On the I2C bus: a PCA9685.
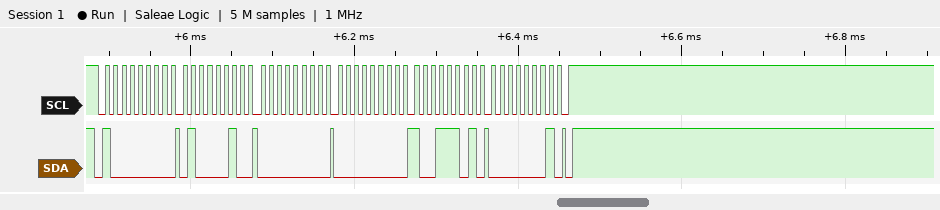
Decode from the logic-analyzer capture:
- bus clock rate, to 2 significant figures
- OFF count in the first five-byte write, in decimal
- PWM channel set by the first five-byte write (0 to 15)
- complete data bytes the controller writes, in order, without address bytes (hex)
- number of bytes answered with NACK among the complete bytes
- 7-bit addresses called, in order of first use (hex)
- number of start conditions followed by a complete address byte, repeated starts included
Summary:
100 kHz
413
15
42 00 00 9D 01
0
0x40
1
